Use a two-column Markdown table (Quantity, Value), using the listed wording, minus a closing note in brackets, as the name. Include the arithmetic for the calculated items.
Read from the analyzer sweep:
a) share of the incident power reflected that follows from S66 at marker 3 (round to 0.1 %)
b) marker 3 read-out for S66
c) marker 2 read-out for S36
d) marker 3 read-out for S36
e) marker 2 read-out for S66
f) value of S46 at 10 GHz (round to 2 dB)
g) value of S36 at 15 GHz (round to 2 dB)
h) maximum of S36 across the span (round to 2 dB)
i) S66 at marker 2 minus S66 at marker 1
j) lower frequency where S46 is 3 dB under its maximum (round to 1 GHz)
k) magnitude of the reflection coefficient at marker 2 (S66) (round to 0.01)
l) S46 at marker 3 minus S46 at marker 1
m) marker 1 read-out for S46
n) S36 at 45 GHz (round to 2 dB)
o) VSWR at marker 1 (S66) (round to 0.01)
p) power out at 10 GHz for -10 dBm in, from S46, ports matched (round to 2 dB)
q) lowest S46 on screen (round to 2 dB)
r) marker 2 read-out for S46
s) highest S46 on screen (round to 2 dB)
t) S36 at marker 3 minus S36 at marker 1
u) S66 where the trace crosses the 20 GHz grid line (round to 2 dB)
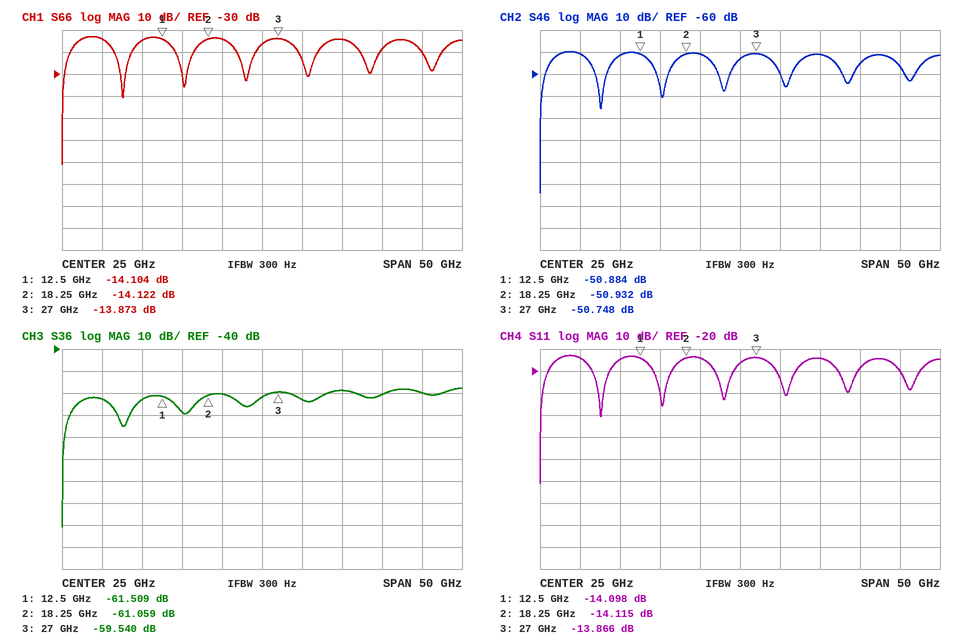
| Quantity | Value |
|---|---|
| share of the incident power reflected that follows from S66 at marker 3 | 10^(-13.873/10) ≈ 4.1 % |
| marker 3 read-out for S66 | -13.873 dB |
| marker 2 read-out for S36 | -61.059 dB |
| marker 3 read-out for S36 | -59.540 dB |
| marker 2 read-out for S66 | -14.122 dB |
| value of S46 at 10 GHz | -52 dB |
| value of S36 at 15 GHz | -68 dB |
| maximum of S36 across the span | -58 dB |
| S66 at marker 2 minus S66 at marker 1 | -14.122 − (-14.104) = -0.018 dB |
| lower frequency where S46 is 3 dB under its maximum | 2 GHz |
| magnitude of the reflection coefficient at marker 2 (S66) | 10^(-14.122/20) ≈ 0.20 |
| S46 at marker 3 minus S46 at marker 1 | -50.748 − (-50.884) = 0.136 dB |
| marker 1 read-out for S46 | -50.884 dB |
| S36 at 45 GHz | -60 dB |
| VSWR at marker 1 (S66) | (1 + 0.1972)/(1 − 0.1972) ≈ 1.49 |
| power out at 10 GHz for -10 dBm in, from S46, ports matched | -10 dBm + (-52 dB) = -62 dBm |
| lowest S46 on screen | -114 dB |
| marker 2 read-out for S46 | -50.932 dB |
| highest S46 on screen | -50 dB |
| S36 at marker 3 minus S36 at marker 1 | -59.54 − (-61.509) = 1.969 dB |
| S66 where the trace crosses the 20 GHz grid line | -14 dB |
